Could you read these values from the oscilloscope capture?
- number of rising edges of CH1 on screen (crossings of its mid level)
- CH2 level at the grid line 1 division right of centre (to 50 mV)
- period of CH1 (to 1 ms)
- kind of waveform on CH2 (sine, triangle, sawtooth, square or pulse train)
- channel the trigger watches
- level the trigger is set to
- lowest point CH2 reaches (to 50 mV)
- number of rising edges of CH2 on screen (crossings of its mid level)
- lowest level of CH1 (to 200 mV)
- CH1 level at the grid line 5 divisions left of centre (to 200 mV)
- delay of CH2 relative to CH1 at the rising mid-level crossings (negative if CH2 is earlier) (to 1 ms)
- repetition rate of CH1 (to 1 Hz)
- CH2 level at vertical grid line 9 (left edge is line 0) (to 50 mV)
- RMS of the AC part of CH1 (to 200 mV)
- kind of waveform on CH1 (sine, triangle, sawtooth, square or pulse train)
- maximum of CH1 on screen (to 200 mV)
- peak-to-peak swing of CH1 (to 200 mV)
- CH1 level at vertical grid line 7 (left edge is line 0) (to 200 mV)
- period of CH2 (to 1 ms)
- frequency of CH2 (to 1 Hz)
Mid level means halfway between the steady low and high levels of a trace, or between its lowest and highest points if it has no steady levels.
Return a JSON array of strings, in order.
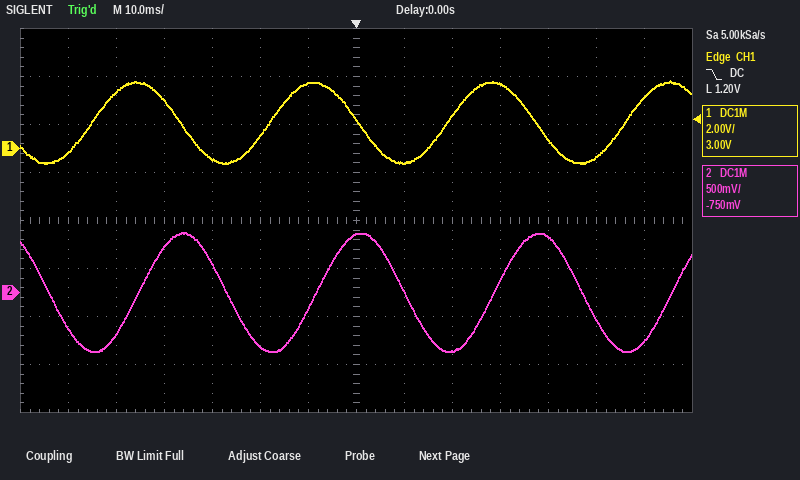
["4", "0 mV", "37 ms", "sine", "CH1", "1.20 V", "-600 mV", "4", "-600 mV", "2.4 V", "+10 ms", "27 Hz", "-600 mV", "1.2 V", "sine", "2.8 V", "3.4 V", "1.2 V", "37 ms", "27 Hz"]
